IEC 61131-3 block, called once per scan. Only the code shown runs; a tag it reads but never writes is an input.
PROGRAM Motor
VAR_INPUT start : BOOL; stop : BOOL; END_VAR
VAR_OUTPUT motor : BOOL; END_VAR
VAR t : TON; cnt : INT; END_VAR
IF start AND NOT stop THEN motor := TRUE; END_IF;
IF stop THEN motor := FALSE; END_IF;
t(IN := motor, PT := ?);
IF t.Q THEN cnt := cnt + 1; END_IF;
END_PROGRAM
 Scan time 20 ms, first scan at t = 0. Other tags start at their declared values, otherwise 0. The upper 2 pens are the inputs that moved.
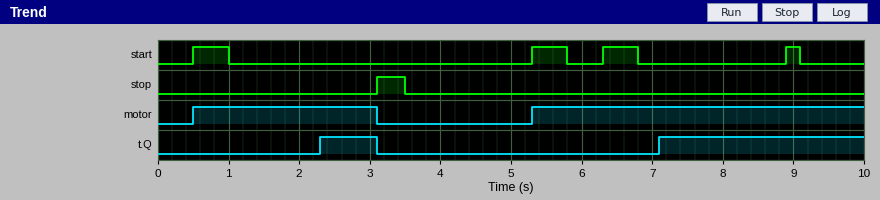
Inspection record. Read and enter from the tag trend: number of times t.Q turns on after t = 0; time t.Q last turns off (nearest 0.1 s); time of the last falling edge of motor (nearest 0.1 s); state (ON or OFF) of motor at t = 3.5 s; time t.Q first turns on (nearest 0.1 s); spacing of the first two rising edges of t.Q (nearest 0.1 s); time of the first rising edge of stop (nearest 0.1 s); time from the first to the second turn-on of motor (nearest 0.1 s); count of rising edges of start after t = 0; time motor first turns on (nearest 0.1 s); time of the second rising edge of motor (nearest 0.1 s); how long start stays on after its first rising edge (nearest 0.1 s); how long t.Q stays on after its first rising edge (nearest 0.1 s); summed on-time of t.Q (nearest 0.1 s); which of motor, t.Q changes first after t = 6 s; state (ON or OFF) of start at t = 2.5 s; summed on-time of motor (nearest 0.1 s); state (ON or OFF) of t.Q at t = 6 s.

2
3.1 s
3.1 s
OFF
2.3 s
4.8 s
3.1 s
4.8 s
4
0.5 s
5.3 s
0.5 s
0.8 s
3.7 s
t.Q
OFF
7.3 s
OFF
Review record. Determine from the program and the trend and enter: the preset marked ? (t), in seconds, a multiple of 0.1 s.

1.8 s
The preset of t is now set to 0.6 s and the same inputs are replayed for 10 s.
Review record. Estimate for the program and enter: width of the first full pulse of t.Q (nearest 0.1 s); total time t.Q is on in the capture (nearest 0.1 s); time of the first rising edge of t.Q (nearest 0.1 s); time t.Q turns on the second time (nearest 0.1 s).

2.0 s
6.1 s
1.1 s
5.9 s
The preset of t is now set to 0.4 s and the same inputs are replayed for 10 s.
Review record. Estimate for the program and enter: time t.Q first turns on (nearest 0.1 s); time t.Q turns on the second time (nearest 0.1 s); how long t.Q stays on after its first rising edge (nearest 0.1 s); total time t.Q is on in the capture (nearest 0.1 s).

0.9 s
5.7 s
2.2 s
6.5 s
